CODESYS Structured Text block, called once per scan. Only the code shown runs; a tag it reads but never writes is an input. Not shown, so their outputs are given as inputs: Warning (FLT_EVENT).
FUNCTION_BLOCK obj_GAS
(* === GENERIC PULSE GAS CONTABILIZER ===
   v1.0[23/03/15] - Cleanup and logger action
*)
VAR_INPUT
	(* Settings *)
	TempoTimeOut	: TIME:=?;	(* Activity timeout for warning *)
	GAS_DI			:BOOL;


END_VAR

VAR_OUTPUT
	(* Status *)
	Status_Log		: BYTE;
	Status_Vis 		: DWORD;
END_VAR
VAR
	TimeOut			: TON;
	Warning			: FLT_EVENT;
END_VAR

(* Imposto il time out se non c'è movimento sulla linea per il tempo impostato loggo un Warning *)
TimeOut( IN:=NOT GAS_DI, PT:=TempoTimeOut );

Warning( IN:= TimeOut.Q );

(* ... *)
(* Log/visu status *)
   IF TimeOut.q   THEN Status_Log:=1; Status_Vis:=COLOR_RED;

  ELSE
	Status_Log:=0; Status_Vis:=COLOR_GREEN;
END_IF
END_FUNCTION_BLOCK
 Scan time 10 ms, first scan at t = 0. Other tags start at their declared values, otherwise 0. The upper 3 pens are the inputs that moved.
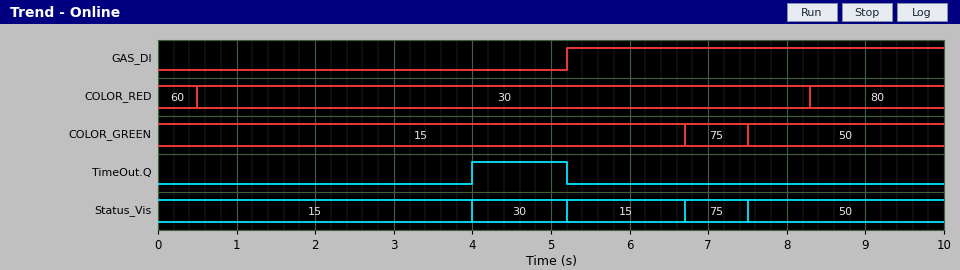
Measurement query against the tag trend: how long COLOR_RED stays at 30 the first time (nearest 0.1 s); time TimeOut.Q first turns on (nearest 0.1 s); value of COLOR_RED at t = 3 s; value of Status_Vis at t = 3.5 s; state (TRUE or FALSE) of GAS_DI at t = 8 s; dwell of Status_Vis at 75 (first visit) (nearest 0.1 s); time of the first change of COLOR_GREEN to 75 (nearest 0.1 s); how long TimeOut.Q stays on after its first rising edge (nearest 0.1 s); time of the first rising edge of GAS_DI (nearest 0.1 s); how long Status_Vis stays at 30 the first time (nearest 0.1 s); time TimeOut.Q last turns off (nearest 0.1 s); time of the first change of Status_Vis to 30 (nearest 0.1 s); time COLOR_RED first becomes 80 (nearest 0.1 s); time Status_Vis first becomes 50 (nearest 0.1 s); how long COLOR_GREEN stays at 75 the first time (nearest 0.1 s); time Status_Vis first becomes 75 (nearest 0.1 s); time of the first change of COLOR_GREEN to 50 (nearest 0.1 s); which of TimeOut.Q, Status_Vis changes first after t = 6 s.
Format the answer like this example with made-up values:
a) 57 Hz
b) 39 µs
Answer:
a) 7.8 s
b) 4.0 s
c) 30
d) 15
e) TRUE
f) 0.8 s
g) 6.7 s
h) 1.2 s
i) 5.2 s
j) 1.2 s
k) 5.2 s
l) 4.0 s
m) 8.3 s
n) 7.5 s
o) 0.8 s
p) 6.7 s
q) 7.5 s
r) Status_Vis
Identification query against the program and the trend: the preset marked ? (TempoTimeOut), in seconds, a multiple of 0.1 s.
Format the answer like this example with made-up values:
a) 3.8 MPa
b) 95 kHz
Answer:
a) 4.0 s
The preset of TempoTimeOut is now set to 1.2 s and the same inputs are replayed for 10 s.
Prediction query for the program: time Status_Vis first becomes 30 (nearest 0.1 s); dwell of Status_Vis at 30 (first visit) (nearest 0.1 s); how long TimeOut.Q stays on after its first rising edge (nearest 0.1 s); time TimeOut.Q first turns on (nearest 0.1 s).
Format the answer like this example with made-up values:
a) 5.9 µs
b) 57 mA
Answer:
a) 1.2 s
b) 4.0 s
c) 4.0 s
d) 1.2 s
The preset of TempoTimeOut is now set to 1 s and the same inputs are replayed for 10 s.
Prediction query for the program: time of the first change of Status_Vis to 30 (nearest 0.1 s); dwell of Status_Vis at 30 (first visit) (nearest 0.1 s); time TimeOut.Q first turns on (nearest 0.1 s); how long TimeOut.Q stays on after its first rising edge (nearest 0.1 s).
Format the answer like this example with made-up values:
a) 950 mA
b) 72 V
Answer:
a) 1.0 s
b) 4.2 s
c) 1.0 s
d) 4.2 s
